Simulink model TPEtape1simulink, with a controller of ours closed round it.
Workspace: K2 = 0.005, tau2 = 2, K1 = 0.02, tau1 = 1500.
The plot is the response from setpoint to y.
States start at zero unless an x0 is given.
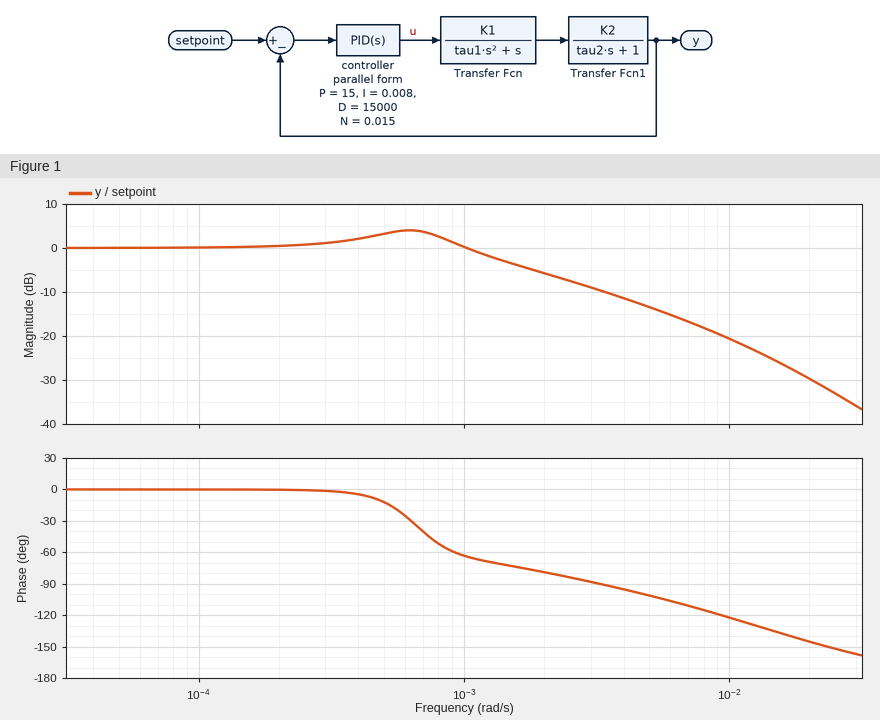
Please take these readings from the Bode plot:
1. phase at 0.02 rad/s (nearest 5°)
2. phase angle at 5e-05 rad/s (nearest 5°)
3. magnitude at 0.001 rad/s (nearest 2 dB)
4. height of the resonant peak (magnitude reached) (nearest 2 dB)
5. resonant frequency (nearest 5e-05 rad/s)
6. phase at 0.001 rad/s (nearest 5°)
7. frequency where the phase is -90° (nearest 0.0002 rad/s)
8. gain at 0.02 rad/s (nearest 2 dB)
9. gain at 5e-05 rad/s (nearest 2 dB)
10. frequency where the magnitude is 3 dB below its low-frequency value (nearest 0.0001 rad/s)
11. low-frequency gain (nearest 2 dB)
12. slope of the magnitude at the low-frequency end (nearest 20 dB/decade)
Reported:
-145°
0°
0 dB
4 dB
0.00060 rad/s
-65°
0.0032 rad/s
-30 dB
0 dB
0.0014 rad/s
0 dB
0 dB/decade
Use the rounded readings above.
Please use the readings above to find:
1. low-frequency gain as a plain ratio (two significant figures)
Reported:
1.0
